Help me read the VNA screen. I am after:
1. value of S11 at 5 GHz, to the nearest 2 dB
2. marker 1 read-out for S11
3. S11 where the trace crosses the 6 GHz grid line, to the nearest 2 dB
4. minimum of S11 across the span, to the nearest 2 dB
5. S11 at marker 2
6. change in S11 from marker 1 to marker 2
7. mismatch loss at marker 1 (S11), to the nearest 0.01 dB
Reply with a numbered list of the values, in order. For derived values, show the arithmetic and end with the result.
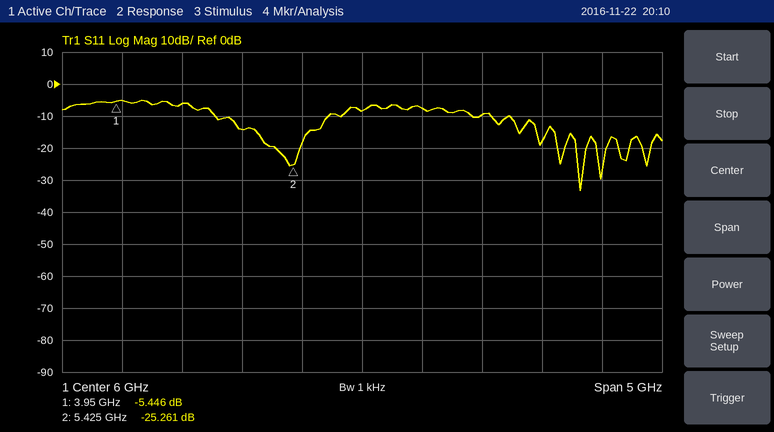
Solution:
1. -14 dB
2. -5.446 dB
3. -8 dB
4. -34 dB
5. -25.261 dB
6. -25.261 − (-5.446) = -19.815 dB
7. −10 log10(1 − 10^(-5.446/10)) ≈ 1.46 dB
